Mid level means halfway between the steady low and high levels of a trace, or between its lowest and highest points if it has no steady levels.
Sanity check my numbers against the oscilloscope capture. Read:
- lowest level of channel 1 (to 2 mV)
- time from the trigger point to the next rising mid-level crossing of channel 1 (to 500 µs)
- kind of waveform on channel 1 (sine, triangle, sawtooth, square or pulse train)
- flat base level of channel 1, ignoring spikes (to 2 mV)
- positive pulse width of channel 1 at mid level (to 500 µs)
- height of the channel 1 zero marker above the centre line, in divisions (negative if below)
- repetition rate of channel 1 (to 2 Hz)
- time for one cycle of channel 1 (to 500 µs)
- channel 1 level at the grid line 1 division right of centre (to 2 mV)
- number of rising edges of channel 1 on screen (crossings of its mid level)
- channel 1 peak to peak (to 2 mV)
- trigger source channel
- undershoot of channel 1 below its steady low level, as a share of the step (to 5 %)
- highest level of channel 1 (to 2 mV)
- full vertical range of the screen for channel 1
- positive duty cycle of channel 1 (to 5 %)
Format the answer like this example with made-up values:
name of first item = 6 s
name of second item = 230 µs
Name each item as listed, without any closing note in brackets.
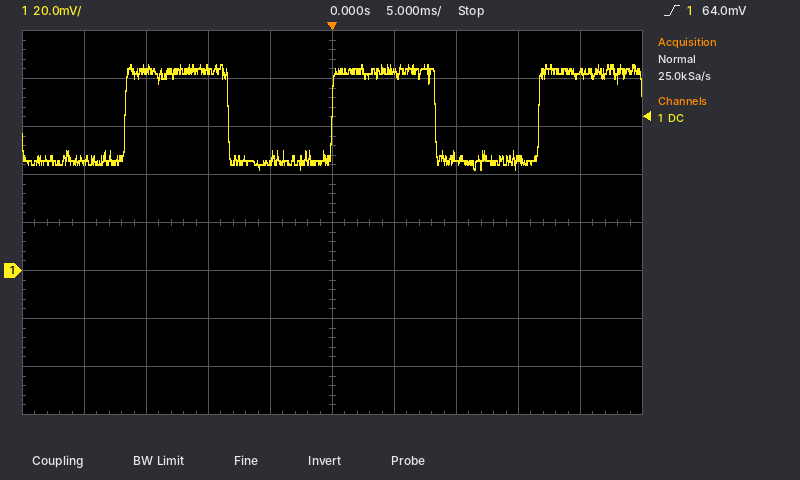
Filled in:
lowest level of channel 1 = 42 mV
time from the trigger point to the next rising mid-level crossing of channel 1 = 16.5 ms
kind of waveform on channel 1 = square
flat base level of channel 1, ignoring spikes = 46 mV
positive pulse width of channel 1 at mid level = 8.5 ms
height of the channel 1 zero marker above the centre line, in divisions = -1.0 div
repetition rate of channel 1 = 60 Hz
time for one cycle of channel 1 = 16.5 ms
channel 1 level at the grid line 1 division right of centre = 82 mV
number of rising edges of channel 1 on screen = 3
channel 1 peak to peak = 44 mV
trigger source channel = channel 1
undershoot of channel 1 below its steady low level, as a share of the step = 10 %
highest level of channel 1 = 86 mV
full vertical range of the screen for channel 1 = 160 mV
positive duty cycle of channel 1 = 50 %
